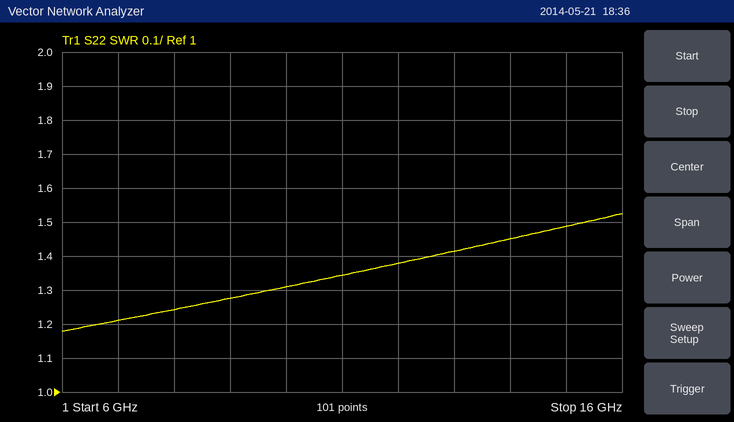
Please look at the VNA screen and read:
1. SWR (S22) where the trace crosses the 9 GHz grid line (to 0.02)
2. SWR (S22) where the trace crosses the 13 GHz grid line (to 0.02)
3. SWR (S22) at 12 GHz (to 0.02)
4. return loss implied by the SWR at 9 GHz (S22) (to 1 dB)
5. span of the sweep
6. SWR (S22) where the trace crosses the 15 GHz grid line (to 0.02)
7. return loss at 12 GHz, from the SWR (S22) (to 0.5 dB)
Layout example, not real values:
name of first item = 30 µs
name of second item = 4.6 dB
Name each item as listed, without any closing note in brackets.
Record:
SWR (S22) where the trace crosses the 9 GHz grid line = 1.28
SWR (S22) where the trace crosses the 13 GHz grid line = 1.42
SWR (S22) at 12 GHz = 1.38
return loss implied by the SWR at 9 GHz (S22) = 18 dB
span of the sweep = 10 GHz
SWR (S22) where the trace crosses the 15 GHz grid line = 1.48
return loss at 12 GHz, from the SWR (S22) = 16.0 dB
